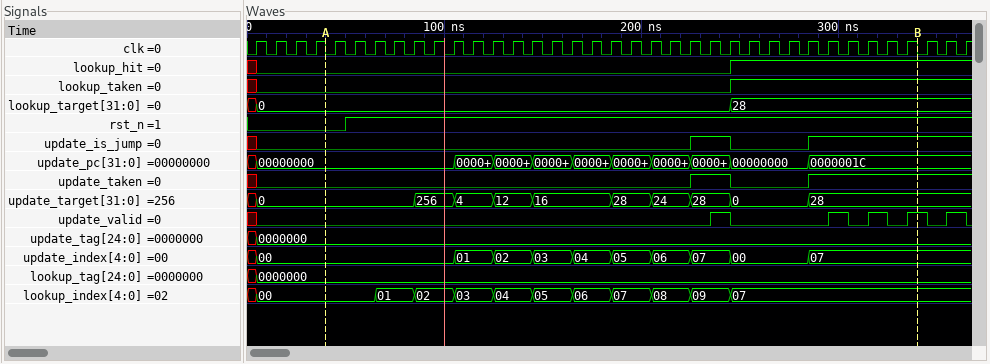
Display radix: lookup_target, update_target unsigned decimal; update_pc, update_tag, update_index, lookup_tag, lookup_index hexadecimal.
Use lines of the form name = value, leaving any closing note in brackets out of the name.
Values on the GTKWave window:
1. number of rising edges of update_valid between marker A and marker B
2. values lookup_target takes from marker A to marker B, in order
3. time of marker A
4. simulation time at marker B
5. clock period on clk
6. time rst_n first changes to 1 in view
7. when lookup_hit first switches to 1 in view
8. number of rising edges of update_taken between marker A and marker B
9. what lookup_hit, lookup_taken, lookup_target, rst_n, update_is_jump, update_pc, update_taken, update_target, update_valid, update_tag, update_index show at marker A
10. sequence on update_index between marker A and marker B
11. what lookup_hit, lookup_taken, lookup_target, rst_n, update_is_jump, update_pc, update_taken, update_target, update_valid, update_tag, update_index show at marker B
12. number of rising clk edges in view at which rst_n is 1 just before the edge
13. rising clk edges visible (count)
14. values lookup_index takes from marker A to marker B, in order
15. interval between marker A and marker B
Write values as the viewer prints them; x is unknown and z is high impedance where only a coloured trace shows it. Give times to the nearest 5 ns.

number of rising edges of update_valid between marker A and marker B = 4
values lookup_target takes from marker A to marker B, in order = 0, 28
time of marker A = 40 ns
simulation time at marker B = 340 ns
clock period on clk = 10 ns
time rst_n first changes to 1 in view = 50 ns
when lookup_hit first switches to 1 in view = 245 ns
number of rising edges of update_taken between marker A and marker B = 2
what lookup_hit, lookup_taken, lookup_target, rst_n, update_is_jump, update_pc, update_taken, update_target, update_valid, update_tag, update_index show at marker A = lookup_hit=0, lookup_taken=0, lookup_target=0, rst_n=0, update_is_jump=0, update_pc=00000000, update_taken=0, update_target=0, update_valid=0, update_tag=0000000, update_index=00
sequence on update_index between marker A and marker B = 00, 01, 02, 03, 04, 05, 06, 07, 00, 07
what lookup_hit, lookup_taken, lookup_target, rst_n, update_is_jump, update_pc, update_taken, update_target, update_valid, update_tag, update_index show at marker B = lookup_hit=1, lookup_taken=1, lookup_target=28, rst_n=1, update_is_jump=1, update_pc=0000001C, update_taken=1, update_target=28, update_valid=1, update_tag=0000000, update_index=07
number of rising clk edges in view at which rst_n is 1 just before the edge = 32
rising clk edges visible = 37
values lookup_index takes from marker A to marker B, in order = 00, 01, 02, 03, 04, 05, 06, 07, 08, 09, 07
interval between marker A and marker B = 300 ns
